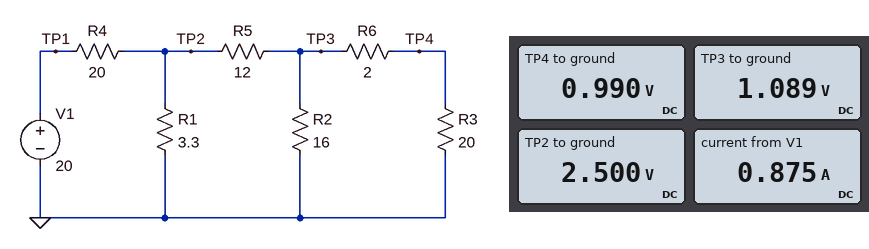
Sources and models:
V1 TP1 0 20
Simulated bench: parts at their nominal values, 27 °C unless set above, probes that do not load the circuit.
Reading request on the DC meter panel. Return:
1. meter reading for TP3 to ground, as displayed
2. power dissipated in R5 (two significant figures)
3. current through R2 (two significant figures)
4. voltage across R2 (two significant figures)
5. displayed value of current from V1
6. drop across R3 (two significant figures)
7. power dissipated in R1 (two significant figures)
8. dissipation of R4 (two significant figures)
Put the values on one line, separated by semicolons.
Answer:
1.089 V; 170 mW; 68 mA; 1.1 V; 0.875 A; 990 mV; 1.9 W; 15 W
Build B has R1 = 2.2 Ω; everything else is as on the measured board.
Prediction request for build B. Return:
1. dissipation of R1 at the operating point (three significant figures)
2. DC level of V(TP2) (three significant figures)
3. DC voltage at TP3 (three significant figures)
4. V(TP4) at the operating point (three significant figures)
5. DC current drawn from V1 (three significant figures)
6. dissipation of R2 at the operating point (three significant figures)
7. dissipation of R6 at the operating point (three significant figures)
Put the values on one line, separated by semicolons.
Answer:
1.49 W; 1.81 V; 790 mV; 718 mV; 909 mA; 39.0 mW; 2.58 mW
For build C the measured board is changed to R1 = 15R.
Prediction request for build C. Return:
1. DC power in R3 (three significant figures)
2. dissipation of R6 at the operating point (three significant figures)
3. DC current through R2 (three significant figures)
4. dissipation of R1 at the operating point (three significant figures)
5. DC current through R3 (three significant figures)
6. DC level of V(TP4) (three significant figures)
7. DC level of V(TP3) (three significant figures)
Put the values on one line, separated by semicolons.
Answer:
293 mW; 29.3 mW; 166 mA; 2.49 W; 121 mA; 2.42 V; 2.66 V
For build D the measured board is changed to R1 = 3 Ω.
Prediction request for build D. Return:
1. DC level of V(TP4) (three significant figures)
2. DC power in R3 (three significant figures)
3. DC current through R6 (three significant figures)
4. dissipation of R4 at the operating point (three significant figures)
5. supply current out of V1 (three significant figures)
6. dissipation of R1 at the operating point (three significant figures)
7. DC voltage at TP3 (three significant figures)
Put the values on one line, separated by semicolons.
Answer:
920 mV; 42.3 mW; 46.0 mA; 15.6 W; 884 mA; 1.80 W; 1.01 V
